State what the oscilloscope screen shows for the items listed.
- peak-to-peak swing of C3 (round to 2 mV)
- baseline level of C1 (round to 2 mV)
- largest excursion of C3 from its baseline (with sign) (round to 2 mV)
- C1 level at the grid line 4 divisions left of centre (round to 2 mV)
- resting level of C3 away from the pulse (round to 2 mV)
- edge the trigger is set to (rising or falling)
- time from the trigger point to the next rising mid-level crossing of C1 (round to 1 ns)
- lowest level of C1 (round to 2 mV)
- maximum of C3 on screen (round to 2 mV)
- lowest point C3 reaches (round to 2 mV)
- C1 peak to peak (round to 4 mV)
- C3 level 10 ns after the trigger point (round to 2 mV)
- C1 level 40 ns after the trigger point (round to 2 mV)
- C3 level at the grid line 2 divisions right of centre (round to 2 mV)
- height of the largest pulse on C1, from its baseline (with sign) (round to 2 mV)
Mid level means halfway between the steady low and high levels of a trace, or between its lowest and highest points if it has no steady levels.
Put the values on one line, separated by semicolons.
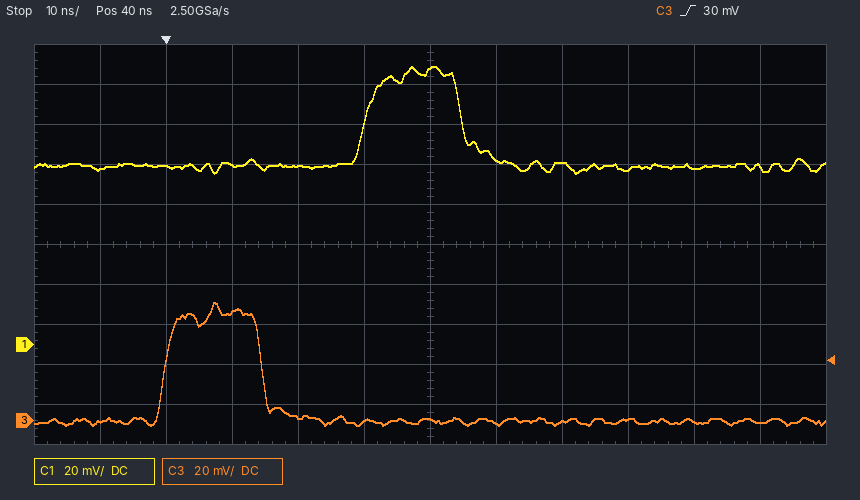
62 mV; 90 mV; +60 mV; 90 mV; 0 mV; rising; 30 ns; 86 mV; 60 mV; -2 mV; 52 mV; 54 mV; 138 mV; 0 mV; +50 mV
